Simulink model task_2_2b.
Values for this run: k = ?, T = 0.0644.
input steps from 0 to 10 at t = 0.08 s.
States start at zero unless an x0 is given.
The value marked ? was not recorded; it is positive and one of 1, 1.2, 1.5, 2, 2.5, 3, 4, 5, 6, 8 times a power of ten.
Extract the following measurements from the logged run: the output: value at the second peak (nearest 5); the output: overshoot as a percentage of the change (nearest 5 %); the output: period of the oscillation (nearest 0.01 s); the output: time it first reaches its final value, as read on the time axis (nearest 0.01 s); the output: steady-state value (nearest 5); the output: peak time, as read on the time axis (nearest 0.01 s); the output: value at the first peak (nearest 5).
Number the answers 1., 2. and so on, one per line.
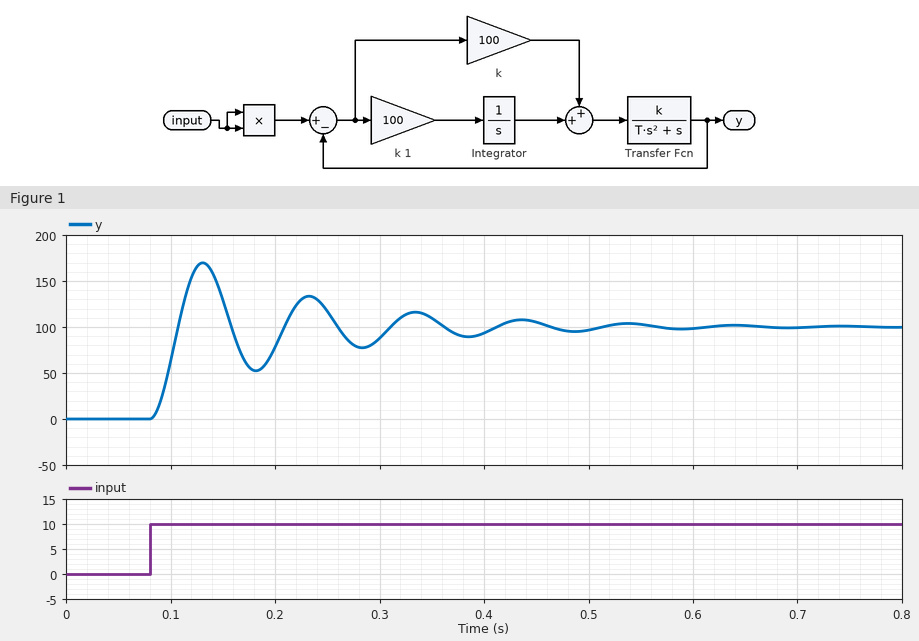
1. 135
2. 70 %
3. 0.10 s
4. 0.11 s
5. 100
6. 0.13 s
7. 170
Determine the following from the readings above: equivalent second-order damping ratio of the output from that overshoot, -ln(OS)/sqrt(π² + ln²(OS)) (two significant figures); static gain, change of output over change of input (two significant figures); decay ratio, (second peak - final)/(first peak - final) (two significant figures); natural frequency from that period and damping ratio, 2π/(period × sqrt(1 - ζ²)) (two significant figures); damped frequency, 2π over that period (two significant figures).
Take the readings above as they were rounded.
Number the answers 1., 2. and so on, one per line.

1. 0.11
2. 10
3. 0.50
4. 63 rad/s
5. 63 rad/s
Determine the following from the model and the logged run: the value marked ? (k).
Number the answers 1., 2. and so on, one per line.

1. 2.5
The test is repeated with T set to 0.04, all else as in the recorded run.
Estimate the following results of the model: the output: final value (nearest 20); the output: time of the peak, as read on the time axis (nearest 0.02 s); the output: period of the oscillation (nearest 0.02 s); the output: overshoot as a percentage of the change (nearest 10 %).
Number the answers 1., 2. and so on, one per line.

1. 100
2. 0.12 s
3. 0.08 s
4. 60 %
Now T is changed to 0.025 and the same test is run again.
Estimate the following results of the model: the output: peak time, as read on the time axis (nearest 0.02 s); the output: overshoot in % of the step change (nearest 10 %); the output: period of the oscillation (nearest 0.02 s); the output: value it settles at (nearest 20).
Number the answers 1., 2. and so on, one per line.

1. 0.12 s
2. 50 %
3. 0.06 s
4. 100
